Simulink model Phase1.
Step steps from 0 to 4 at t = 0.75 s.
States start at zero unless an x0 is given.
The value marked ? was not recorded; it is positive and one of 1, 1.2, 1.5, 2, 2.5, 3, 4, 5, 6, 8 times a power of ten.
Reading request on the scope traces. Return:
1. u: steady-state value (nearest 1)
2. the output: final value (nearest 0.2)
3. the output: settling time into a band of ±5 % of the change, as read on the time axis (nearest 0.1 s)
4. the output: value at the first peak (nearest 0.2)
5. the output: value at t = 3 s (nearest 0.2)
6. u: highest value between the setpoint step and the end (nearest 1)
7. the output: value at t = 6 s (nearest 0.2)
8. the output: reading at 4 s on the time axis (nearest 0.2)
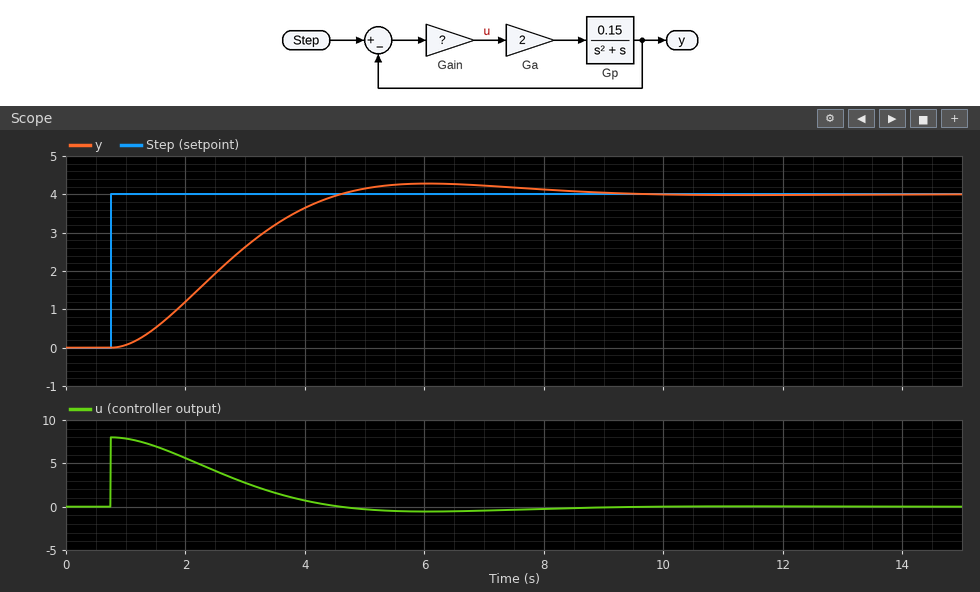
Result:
0
4.0
7.3 s
4.2
2.6
8
4.2
3.6
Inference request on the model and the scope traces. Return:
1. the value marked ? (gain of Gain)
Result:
2
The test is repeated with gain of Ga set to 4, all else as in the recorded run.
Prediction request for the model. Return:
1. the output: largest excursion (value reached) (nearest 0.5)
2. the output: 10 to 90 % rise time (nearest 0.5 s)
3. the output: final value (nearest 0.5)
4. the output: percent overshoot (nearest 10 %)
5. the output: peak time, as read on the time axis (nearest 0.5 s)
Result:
5.0
1.5 s
4.0
20 %
4.0 s
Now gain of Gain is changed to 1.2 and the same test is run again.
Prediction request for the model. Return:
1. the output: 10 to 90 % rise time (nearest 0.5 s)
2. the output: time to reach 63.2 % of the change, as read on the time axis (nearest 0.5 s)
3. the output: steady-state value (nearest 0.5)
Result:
4.5 s
4.0 s
4.0
